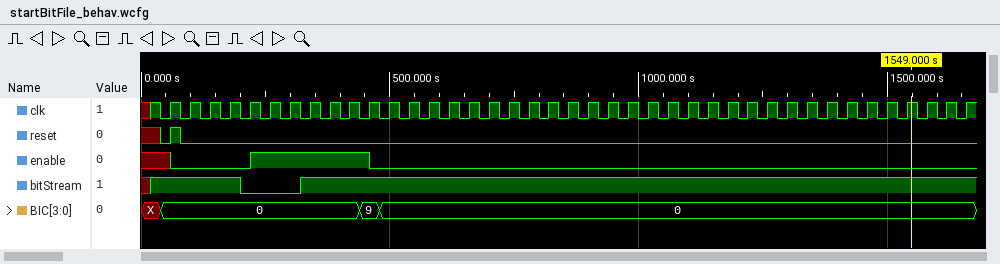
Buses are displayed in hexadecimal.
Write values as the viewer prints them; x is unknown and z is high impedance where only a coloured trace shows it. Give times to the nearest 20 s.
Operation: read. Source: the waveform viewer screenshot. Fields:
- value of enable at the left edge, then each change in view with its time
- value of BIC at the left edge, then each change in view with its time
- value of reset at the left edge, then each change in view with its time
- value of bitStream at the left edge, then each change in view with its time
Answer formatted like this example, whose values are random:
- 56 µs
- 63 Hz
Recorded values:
- x, 0 at 60 s, 1 at 220 s, 0 at 460 s
- X, 0 at 40 s, 9 at 440 s, 0 at 480 s
- x, 0 at 40 s, 1 at 60 s, 0 at 80 s
- x, 1 at 20 s, 0 at 200 s, 1 at 320 s
